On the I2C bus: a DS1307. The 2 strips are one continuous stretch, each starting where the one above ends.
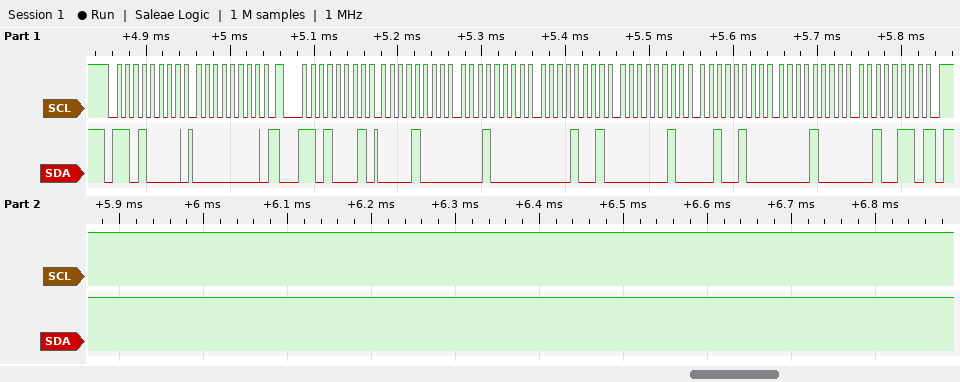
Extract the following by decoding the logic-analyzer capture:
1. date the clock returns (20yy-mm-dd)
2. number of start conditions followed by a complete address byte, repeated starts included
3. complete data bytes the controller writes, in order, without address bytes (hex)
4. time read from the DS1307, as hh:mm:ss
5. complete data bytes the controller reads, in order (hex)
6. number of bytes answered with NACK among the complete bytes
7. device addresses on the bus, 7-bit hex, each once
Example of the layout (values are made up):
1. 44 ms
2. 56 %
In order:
1. 2026-08-24
2. 2
3. 00
4. 09:10:08
5. 08 10 09 02 24 08 26
6. 1
7. 0x68
